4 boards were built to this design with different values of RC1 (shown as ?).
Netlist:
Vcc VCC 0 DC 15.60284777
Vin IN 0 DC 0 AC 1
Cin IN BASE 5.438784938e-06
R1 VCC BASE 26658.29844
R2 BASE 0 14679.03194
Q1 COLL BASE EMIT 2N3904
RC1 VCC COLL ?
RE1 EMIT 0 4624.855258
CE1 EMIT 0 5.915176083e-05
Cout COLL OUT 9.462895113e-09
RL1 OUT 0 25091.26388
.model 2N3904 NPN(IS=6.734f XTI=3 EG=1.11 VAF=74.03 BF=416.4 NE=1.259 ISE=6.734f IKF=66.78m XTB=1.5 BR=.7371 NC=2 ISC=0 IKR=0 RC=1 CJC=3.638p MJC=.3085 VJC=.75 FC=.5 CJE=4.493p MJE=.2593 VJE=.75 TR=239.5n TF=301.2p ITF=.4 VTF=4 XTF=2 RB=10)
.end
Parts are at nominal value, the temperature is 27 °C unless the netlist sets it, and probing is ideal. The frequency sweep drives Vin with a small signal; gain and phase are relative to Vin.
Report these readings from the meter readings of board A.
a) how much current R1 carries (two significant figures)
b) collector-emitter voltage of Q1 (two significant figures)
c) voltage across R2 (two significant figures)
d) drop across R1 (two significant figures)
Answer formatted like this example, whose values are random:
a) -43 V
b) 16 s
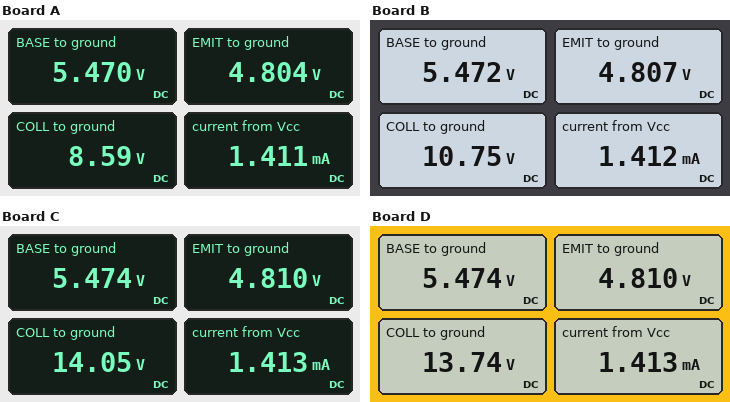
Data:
a) 380 µA
b) 3.8 V
c) 5.5 V
d) 10 V
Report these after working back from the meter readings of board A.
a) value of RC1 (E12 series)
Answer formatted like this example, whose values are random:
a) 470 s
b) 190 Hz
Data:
a) 6.8 kΩ
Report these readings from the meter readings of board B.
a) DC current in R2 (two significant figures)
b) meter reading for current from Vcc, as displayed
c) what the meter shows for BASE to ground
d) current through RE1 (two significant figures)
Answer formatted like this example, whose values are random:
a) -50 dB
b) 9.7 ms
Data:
a) 370 µA
b) 1.412 mA
c) 5.472 V
d) 1.0 mA
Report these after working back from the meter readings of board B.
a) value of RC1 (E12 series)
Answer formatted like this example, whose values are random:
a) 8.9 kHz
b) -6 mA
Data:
a) 4.7 kΩ
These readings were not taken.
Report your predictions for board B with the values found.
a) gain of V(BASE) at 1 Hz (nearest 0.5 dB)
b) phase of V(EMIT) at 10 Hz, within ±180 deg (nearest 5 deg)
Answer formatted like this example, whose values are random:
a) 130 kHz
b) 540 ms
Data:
a) -10.5 dB
b) 10 deg
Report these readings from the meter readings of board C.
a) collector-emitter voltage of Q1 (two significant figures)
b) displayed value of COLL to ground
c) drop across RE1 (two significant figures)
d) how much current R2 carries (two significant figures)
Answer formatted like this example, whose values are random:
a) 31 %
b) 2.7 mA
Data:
a) 9.2 V
b) 14.05 V
c) 4.8 V
d) 370 µA
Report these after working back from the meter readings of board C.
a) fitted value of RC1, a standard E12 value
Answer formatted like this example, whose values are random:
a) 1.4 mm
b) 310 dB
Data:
a) 1.5 kΩ
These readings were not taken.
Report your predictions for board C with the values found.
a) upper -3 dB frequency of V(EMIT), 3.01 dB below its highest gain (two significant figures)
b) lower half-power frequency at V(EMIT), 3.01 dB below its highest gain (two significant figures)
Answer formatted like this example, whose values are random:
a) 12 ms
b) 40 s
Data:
a) 120 Hz
b) 2.8 Hz
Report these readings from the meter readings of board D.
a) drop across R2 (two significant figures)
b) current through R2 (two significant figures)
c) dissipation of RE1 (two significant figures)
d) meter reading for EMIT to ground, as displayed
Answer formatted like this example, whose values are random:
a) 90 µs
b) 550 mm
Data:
a) 5.5 V
b) 370 µA
c) 5.0 mW
d) 4.810 V
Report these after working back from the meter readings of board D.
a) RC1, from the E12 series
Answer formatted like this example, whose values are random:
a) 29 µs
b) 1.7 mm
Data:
a) 1.8 kΩ
